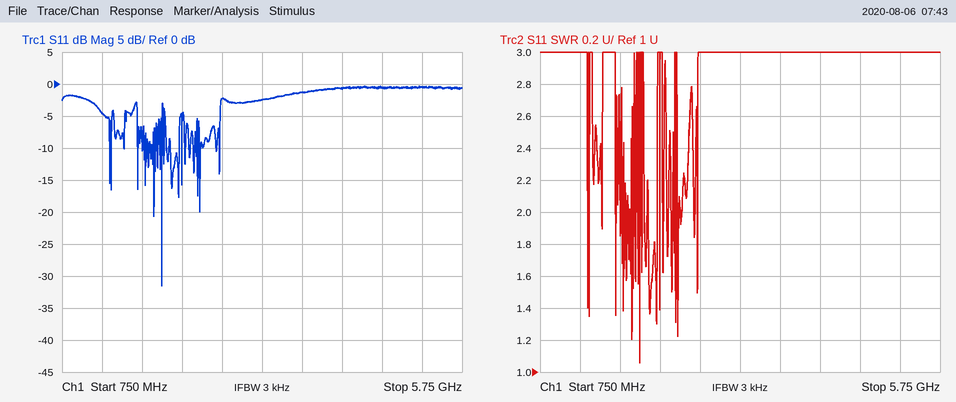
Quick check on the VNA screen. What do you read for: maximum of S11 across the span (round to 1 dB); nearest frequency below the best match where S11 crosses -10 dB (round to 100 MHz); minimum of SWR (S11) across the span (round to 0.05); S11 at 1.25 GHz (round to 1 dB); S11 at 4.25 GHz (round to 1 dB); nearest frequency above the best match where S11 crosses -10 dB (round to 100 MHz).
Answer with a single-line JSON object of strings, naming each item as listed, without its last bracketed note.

{"maximum of S11 across the span": "0 dB", "nearest frequency below the best match where S11 crosses -10 dB": "2.0 GHz", "minimum of SWR (S11) across the span": "1.05", "S11 at 1.25 GHz": "-5 dB", "S11 at 4.25 GHz": "-1 dB", "nearest frequency above the best match where S11 crosses -10 dB": "2.0 GHz"}
